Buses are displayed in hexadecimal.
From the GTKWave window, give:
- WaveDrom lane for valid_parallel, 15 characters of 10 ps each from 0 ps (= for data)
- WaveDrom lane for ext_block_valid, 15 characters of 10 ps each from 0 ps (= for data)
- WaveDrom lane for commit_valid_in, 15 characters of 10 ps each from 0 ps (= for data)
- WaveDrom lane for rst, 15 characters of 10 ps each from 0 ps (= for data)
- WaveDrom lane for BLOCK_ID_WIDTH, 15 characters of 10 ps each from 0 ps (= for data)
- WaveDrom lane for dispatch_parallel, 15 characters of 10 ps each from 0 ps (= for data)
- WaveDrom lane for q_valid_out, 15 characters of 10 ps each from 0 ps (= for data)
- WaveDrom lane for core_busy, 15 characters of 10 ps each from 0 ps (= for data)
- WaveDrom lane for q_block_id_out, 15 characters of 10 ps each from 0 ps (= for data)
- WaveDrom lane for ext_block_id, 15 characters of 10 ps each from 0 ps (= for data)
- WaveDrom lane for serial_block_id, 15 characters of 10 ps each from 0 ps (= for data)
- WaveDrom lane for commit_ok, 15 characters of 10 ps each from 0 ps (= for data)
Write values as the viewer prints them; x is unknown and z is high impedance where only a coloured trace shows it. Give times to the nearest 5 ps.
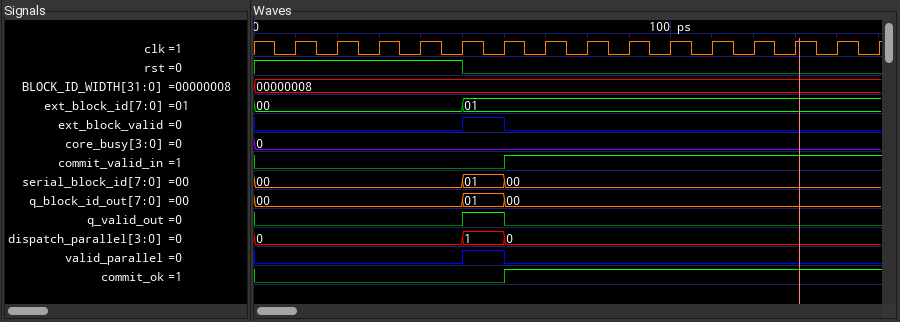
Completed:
{name: 'valid_parallel', wave: '0....10........'}
{name: 'ext_block_valid', wave: '0....10........'}
{name: 'commit_valid_in', wave: '0.....1........'}
{name: 'rst', wave: '1....0.........'}
{name: 'BLOCK_ID_WIDTH', wave: '=..............', data: '00000008'}
{name: 'dispatch_parallel', wave: '=....==........', data: '0 1 0'}
{name: 'q_valid_out', wave: '0....10........'}
{name: 'core_busy', wave: '=..............', data: '0'}
{name: 'q_block_id_out', wave: '=....==........', data: '00 01 00'}
{name: 'ext_block_id', wave: '=....=.........', data: '00 01'}
{name: 'serial_block_id', wave: '=....==........', data: '00 01 00'}
{name: 'commit_ok', wave: '0.....1........'}
